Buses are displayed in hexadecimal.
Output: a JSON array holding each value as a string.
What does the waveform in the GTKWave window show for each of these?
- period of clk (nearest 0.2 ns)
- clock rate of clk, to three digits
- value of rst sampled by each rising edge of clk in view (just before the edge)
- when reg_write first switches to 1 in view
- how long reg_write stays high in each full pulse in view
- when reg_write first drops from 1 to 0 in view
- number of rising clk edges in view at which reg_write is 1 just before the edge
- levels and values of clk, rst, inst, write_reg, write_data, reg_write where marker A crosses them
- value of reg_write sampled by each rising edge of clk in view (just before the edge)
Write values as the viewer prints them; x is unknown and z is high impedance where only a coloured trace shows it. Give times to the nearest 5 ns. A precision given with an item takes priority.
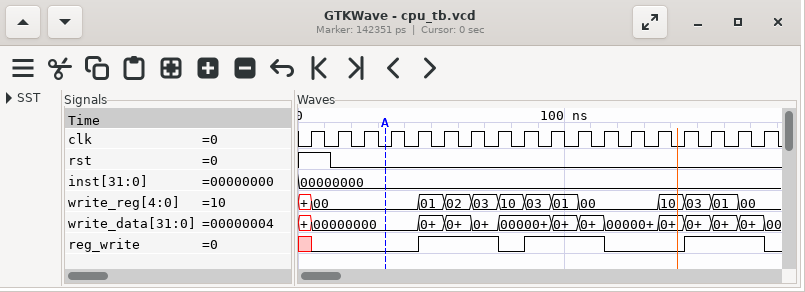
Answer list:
["10 ns", "100 MHz", "1 0 0 0 0 0 0 0 0 0 0 0 0 0 0 0 0 0", "45 ns", "30 ns, 30 ns, 30 ns", "75 ns", "9", "clk=0, rst=0, inst=00000000, write_reg=00, write_data=00000000, reg_write=0", "x 0 0 0 0 1 1 1 0 1 1 1 0 0 0 1 1 1"]
